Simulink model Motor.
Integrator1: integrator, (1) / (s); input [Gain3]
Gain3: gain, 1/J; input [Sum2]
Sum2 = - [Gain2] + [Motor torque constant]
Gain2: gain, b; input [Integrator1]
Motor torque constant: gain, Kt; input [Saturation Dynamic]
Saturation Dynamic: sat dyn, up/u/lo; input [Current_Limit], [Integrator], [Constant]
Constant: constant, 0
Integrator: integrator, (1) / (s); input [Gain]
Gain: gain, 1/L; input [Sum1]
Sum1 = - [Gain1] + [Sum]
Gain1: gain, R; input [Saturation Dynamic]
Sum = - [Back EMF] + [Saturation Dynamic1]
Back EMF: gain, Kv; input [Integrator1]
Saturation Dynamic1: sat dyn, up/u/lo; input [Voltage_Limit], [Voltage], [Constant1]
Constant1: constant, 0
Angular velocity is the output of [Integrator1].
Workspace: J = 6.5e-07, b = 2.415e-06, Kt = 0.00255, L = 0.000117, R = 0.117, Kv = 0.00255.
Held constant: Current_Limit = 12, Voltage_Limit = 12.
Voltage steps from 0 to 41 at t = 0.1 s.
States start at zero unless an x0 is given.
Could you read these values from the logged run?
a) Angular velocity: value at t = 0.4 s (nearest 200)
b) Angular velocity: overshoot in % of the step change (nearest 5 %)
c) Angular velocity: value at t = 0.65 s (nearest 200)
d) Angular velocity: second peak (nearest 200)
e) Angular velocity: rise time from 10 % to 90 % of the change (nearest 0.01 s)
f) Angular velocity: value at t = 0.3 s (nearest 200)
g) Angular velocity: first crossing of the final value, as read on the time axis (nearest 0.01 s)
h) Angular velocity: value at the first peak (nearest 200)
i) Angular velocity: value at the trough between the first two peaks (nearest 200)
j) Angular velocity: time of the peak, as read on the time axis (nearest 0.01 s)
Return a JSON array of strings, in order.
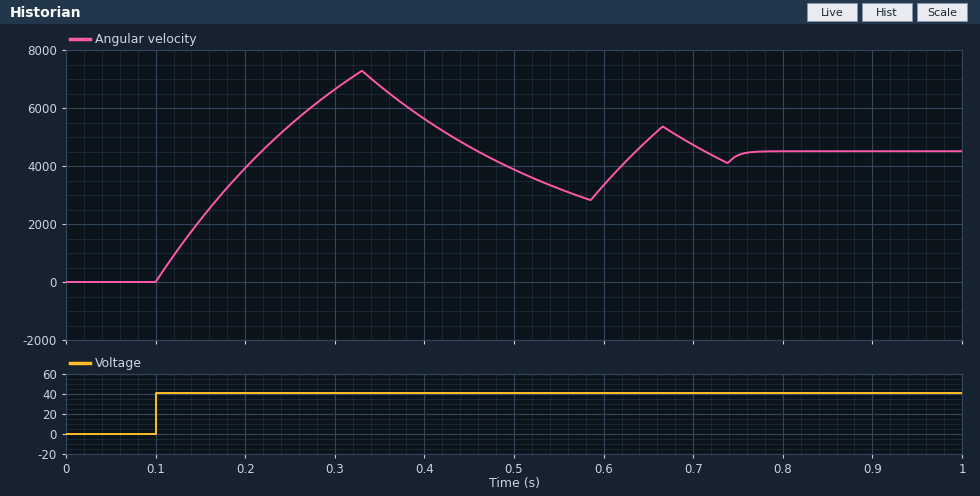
["5600", "60 %", "5000", "5400", "0.09 s", "6600", "0.22 s", "7200", "2800", "0.33 s"]
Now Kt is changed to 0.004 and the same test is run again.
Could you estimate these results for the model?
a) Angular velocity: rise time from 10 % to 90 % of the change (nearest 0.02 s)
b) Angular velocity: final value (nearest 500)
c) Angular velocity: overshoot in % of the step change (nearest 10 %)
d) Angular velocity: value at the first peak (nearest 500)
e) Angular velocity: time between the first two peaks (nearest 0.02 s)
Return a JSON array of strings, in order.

["0.06 s", "4500", "70 %", "7500", "0.34 s"]
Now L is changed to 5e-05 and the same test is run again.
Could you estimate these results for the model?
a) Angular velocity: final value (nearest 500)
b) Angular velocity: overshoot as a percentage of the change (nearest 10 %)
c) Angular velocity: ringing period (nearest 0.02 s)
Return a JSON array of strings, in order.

["4500", "60 %", "0.34 s"]
